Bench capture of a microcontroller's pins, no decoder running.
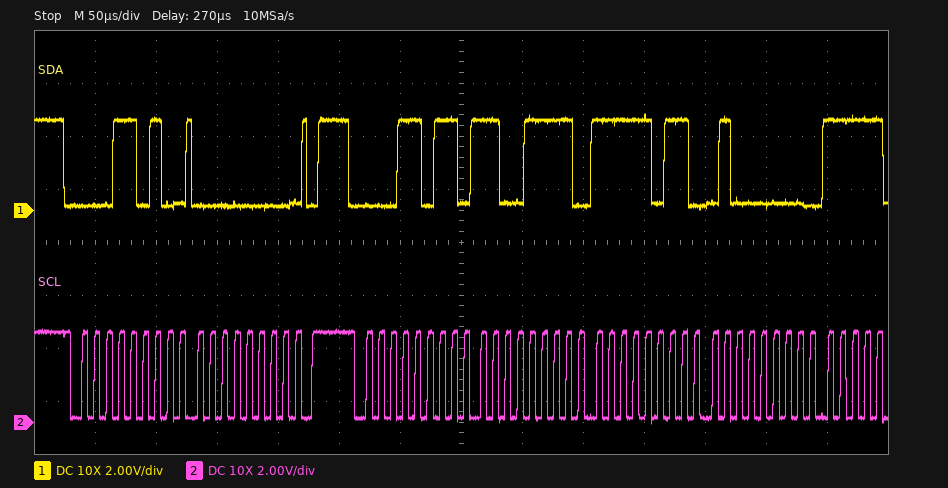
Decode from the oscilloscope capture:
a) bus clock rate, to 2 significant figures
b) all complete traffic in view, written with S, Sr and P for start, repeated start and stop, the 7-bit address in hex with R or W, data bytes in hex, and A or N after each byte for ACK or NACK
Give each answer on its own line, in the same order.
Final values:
100 kHz
S 0DW A 00 A P S 0DR A CF A FB A 40 A
